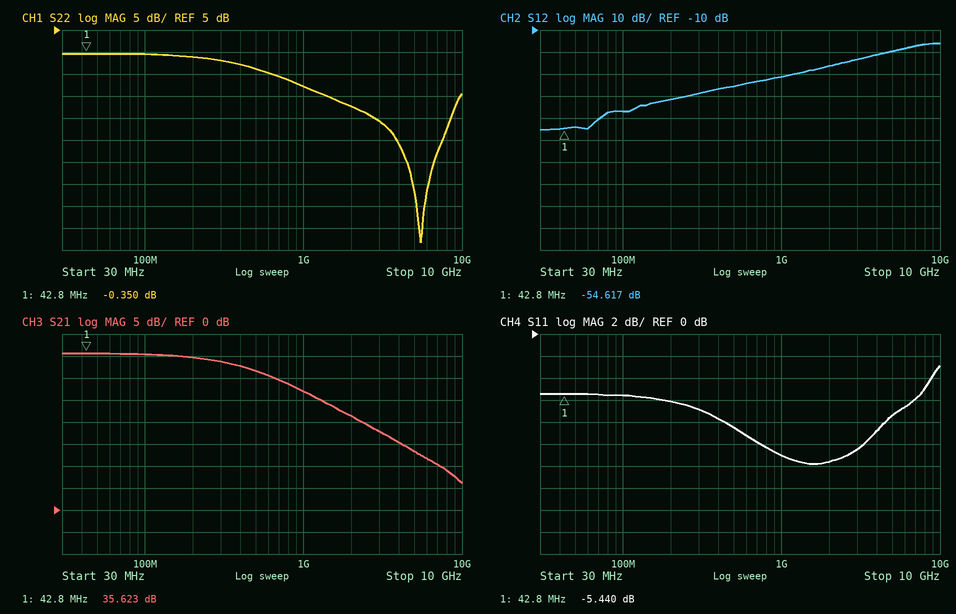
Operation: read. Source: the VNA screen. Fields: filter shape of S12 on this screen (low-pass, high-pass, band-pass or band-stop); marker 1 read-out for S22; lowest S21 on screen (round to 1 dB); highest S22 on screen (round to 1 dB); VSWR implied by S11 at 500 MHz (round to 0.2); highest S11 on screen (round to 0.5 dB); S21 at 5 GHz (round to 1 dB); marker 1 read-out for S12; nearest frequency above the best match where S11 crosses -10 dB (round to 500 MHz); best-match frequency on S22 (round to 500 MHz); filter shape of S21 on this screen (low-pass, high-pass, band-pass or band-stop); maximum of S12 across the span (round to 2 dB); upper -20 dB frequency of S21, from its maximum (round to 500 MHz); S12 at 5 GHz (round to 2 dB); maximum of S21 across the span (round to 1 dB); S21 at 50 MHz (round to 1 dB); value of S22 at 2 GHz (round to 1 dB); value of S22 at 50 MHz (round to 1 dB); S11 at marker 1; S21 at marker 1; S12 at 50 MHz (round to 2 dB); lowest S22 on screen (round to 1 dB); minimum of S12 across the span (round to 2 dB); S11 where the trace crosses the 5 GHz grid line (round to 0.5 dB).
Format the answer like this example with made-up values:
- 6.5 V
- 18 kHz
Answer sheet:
- high-pass
- -0.350 dB
- 6 dB
- 0 dB
- 2.2
- -3.0 dB
- 13 dB
- -54.617 dB
- 3.5 GHz
- 5.5 GHz
- low-pass
- -16 dB
- 4.0 GHz
- -20 dB
- 36 dB
- 36 dB
- -12 dB
- 0 dB
- -5.440 dB
- 35.623 dB
- -54 dB
- -43 dB
- -56 dB
- -7.5 dB
